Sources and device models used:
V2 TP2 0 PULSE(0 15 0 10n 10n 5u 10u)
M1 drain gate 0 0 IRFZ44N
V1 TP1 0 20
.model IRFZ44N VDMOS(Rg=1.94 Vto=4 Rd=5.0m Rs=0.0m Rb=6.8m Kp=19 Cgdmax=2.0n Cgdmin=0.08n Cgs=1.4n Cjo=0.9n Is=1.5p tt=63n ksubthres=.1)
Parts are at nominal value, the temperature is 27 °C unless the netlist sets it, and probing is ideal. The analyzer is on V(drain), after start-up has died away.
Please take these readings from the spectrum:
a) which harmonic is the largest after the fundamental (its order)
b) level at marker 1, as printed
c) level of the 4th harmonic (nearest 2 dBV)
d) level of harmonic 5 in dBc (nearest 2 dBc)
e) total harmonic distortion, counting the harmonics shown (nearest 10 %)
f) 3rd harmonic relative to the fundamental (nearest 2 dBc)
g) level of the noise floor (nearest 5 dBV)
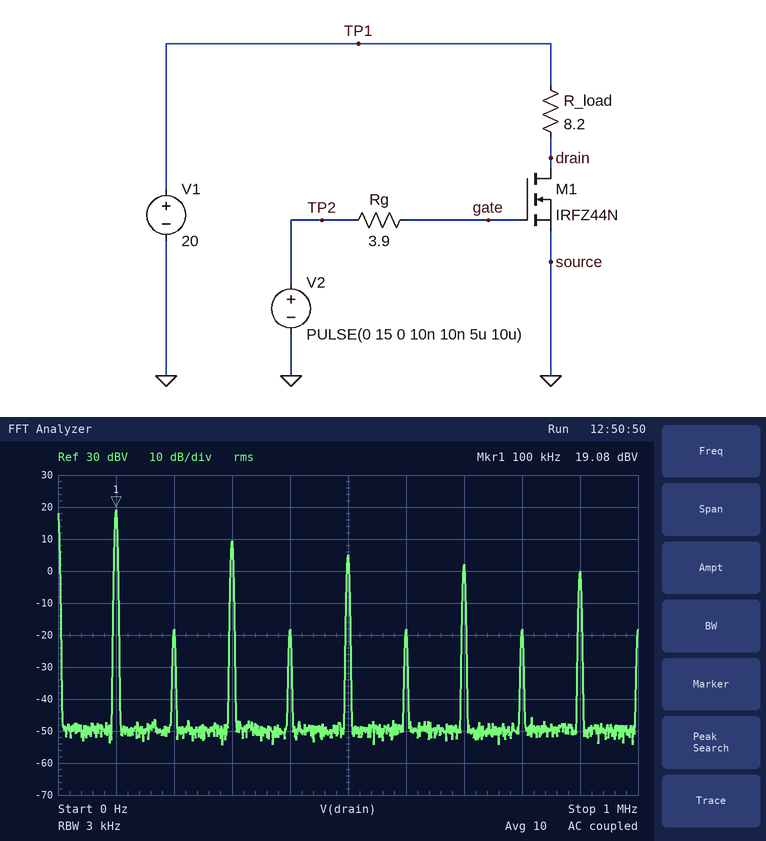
3
19.08 dBV
-18 dBV
-14 dBc
40 %
-10 dBc
-50 dBV
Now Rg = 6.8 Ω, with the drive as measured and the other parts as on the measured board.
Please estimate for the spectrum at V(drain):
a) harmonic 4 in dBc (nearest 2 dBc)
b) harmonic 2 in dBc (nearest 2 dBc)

-34 dBc
-34 dBc
